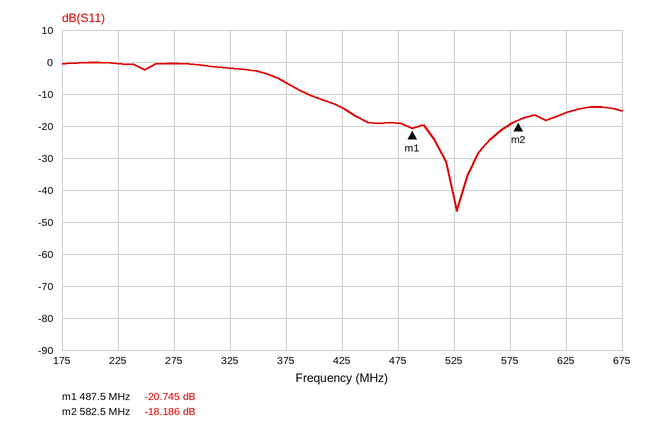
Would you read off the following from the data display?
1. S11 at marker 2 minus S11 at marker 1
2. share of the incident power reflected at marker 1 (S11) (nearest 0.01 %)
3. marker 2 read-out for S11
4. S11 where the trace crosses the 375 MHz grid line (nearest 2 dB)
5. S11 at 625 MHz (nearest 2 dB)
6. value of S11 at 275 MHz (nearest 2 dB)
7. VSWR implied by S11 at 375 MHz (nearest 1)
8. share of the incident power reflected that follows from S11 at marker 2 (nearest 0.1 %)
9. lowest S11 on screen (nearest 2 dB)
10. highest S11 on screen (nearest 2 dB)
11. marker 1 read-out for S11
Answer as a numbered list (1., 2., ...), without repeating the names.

1. 2.559 dB
2. 0.84 %
3. -18.186 dB
4. -6 dB
5. -16 dB
6. 0 dB
7. 3
8. 1.5 %
9. -46 dB
10. 0 dB
11. -20.745 dB
